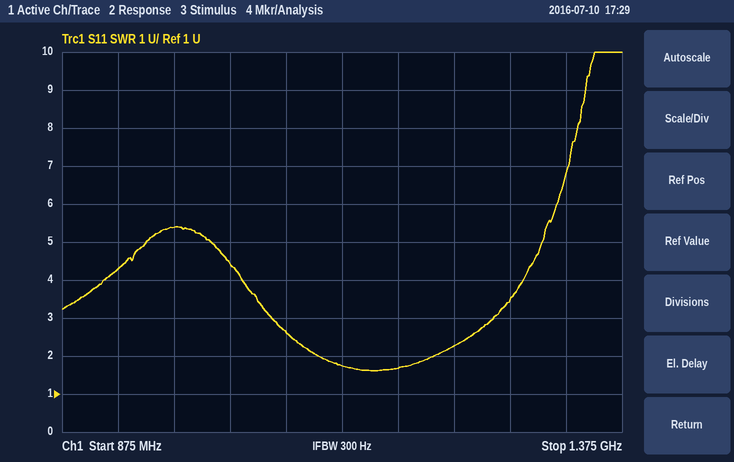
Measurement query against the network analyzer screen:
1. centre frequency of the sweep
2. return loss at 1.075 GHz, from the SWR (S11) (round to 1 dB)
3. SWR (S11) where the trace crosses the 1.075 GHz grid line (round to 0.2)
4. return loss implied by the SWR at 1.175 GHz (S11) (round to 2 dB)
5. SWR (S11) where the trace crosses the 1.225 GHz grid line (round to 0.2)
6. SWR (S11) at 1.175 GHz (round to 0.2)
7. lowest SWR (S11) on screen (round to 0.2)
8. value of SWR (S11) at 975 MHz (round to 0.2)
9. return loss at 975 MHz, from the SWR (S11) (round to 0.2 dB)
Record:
1.125 GHz
7 dB
2.6
12 dB
2.2
1.6
1.6
5.4
3.2 dB
